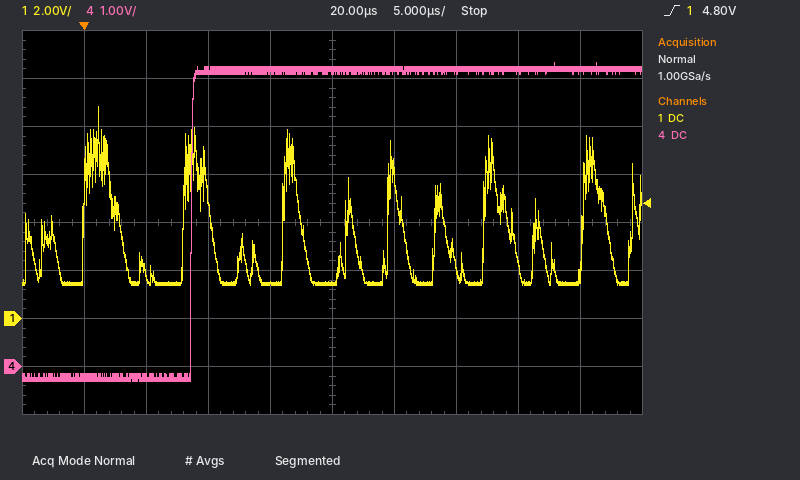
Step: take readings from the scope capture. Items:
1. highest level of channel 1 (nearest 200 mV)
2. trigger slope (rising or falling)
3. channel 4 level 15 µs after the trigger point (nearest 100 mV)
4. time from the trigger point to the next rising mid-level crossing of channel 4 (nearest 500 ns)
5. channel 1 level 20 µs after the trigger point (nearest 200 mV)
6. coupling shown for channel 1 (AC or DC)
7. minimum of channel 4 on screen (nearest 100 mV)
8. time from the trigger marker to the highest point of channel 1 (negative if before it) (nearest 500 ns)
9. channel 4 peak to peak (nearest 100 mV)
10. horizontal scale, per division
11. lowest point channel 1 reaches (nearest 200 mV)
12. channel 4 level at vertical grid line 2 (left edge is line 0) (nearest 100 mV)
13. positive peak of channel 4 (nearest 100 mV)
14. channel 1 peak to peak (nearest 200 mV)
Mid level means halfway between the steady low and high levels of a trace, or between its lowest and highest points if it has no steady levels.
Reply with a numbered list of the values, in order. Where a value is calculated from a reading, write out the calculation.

1. 8.8 V
2. rising
3. 6.2 V
4. 8.5 µs
5. 1.4 V
6. DC
7. -300 mV
8. +1.0 µs
9. 6.3 V − (-300 mV) = 6.6 V
10. 5 µs
11. 1.4 V
12. -200 mV
13. 6.3 V
14. 8.8 V − (1.4 V) = 7.4 V
